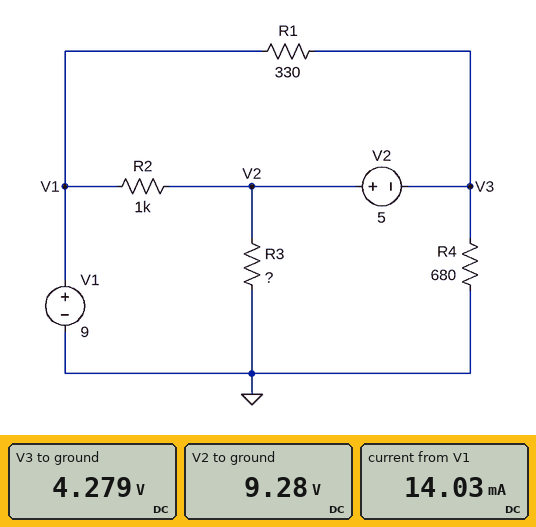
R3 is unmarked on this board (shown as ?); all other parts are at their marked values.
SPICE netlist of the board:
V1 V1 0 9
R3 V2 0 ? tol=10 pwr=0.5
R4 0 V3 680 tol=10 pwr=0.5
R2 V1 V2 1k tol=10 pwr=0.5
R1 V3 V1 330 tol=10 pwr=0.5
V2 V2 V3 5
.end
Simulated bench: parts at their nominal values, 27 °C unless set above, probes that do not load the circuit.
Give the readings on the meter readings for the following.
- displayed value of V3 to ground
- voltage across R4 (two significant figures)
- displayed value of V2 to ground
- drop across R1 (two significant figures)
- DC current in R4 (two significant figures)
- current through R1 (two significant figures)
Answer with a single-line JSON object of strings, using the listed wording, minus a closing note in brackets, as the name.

{"displayed value of V3 to ground": "4.279 V", "voltage across R4": "4.3 V", "displayed value of V2 to ground": "9.28 V", "drop across R1": "4.7 V", "DC current in R4": "6.3 mA", "current through R1": "14 mA"}
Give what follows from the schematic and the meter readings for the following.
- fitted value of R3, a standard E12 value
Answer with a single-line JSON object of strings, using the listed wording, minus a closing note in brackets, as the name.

{"fitted value of R3, a standard E12 value": "1.2 kΩ"}
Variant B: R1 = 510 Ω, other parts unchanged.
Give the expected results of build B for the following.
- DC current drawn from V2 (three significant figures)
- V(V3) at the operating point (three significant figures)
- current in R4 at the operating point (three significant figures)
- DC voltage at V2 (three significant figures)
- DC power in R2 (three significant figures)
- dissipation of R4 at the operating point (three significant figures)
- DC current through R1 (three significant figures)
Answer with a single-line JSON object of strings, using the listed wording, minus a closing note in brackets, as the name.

{"DC current drawn from V2": "6.25 mA", "V(V3) at the operating point": "3.32 V", "current in R4 at the operating point": "4.88 mA", "DC voltage at V2": "8.32 V", "DC power in R2": "462 µW", "dissipation of R4 at the operating point": "16.2 mW", "DC current through R1": "11.1 mA"}
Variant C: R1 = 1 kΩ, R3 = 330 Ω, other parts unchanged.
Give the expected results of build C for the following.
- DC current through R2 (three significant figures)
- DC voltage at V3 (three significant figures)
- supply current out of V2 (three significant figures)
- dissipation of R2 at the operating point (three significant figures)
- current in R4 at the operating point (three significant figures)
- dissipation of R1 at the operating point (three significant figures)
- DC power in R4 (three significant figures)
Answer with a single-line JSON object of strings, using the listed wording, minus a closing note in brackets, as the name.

{"DC current through R2": "4.33 mA", "DC voltage at V3": "-331 mV", "supply current out of V2": "9.82 mA", "dissipation of R2 at the operating point": "18.8 mW", "current in R4 at the operating point": "487 µA", "dissipation of R1 at the operating point": "87.1 mW", "DC power in R4": "161 µW"}
